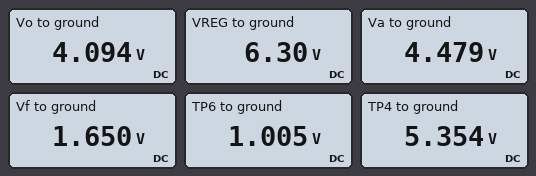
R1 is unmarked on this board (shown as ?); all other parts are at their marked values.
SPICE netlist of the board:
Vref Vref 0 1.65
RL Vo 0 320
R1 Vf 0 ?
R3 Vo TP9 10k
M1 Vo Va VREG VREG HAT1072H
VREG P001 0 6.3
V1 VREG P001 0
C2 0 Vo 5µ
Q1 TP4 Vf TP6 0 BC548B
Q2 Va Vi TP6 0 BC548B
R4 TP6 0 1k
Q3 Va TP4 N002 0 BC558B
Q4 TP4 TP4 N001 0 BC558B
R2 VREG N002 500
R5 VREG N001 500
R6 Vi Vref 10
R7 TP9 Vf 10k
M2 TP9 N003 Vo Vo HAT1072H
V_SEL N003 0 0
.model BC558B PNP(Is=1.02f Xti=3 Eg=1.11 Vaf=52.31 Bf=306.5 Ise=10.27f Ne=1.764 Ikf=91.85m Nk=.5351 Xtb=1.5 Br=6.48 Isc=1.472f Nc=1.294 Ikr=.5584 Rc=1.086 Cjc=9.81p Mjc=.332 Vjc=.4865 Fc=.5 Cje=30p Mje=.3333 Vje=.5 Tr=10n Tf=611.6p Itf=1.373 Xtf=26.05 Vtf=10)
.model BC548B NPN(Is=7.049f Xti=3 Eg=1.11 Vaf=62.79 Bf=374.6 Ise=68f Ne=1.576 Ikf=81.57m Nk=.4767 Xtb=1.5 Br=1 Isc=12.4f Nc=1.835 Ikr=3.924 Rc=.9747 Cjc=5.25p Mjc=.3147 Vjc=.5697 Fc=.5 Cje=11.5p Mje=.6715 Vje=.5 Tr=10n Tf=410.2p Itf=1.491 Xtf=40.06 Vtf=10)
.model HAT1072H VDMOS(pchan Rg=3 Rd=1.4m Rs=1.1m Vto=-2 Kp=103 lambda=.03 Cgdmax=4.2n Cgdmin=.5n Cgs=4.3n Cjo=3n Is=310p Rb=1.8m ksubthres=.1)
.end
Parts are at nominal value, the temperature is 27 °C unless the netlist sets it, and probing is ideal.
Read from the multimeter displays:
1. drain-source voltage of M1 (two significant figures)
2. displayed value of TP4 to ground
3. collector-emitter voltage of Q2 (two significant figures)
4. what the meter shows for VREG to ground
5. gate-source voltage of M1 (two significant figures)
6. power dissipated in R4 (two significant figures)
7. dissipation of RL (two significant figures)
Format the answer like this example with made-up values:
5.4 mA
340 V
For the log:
-2.2 V
5.354 V
3.5 V
6.30 V
-1.8 V
1.0 mW
52 mW
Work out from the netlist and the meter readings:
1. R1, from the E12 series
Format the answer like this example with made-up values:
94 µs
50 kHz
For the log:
6.8 kΩ
